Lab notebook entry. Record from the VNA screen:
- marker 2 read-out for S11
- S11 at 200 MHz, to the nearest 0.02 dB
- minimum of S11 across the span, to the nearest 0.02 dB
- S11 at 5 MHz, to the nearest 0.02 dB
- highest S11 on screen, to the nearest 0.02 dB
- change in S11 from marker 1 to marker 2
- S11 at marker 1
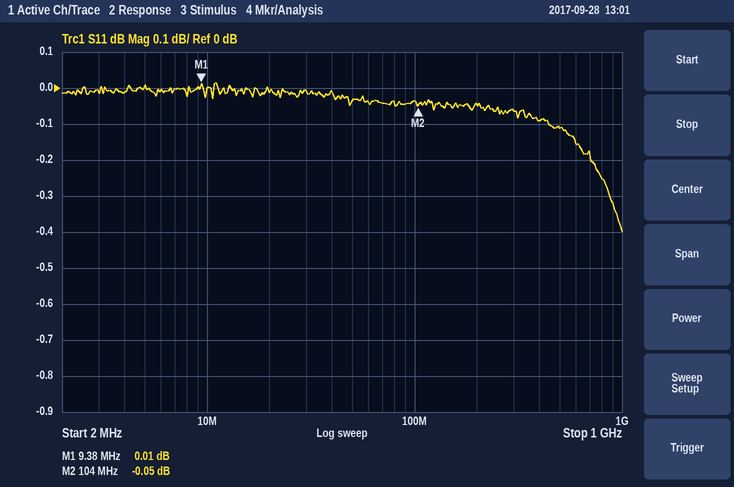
-0.05 dB
-0.04 dB
-0.40 dB
0.00 dB
0.02 dB
-0.06 dB
0.01 dB
